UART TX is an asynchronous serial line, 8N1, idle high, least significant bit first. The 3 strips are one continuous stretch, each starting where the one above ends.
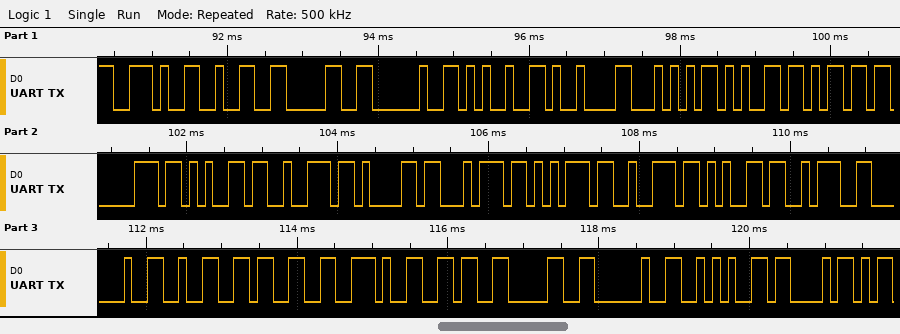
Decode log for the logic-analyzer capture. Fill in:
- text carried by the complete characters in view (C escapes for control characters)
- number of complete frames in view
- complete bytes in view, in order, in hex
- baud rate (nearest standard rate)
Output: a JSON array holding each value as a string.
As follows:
["\".20 %\\tTemperature: 23.60 *C\"", "27", "2E 32 30 20 25 09 54 65 6D 70 65 72 61 74 75 72 65 3A 20 32 33 2E 36 30 20 2A 43", "9600 baud"]
